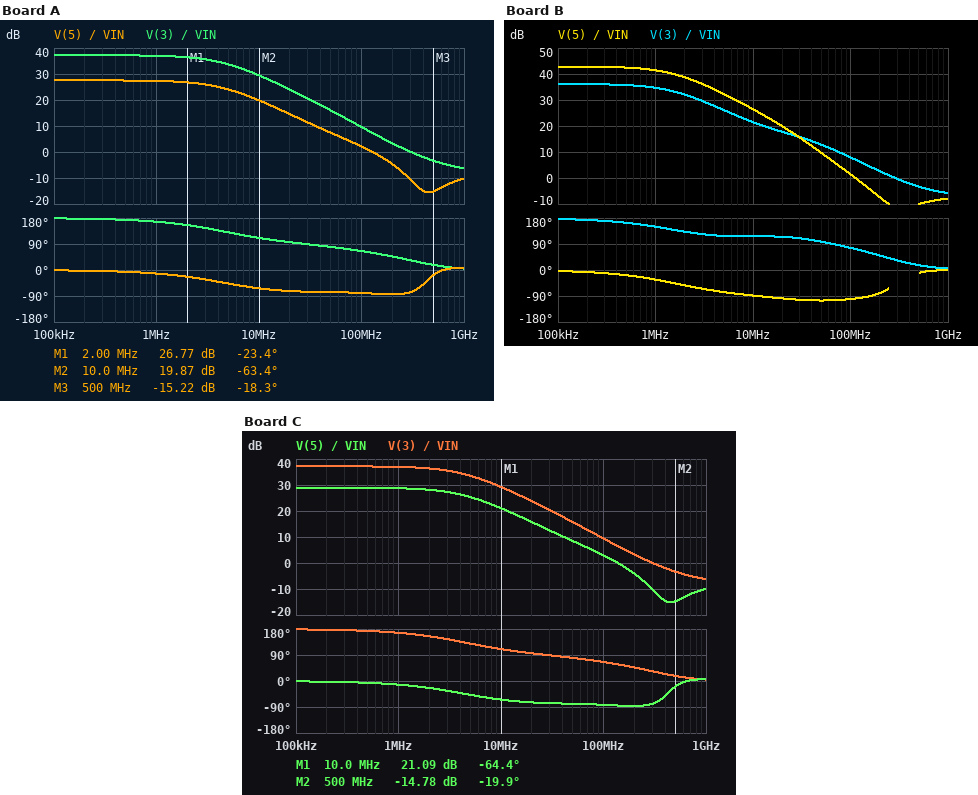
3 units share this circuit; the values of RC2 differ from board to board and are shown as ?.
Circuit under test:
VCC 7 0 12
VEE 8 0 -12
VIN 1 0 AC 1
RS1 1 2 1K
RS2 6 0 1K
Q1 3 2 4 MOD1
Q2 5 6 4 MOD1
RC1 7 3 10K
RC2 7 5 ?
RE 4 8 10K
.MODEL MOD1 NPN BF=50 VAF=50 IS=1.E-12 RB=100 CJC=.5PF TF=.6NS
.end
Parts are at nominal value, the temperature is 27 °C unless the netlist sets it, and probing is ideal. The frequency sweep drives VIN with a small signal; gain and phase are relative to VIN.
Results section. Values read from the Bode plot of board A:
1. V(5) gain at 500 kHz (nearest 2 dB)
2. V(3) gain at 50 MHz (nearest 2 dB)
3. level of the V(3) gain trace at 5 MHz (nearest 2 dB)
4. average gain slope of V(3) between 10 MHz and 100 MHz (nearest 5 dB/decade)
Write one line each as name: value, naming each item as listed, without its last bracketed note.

V(5) gain at 500 kHz: 28 dB
V(3) gain at 50 MHz: 16 dB
level of the V(3) gain trace at 5 MHz: 34 dB
average gain slope of V(3) between 10 MHz and 100 MHz: -20 dB/decade
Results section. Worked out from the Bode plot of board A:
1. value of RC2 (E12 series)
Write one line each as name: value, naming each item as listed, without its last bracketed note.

value of RC2: 3.3 kΩ
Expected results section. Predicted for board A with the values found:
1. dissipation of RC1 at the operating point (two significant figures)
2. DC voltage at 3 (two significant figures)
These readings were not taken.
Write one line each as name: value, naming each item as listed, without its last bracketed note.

dissipation of RC1 at the operating point: 3.0 mW
DC voltage at 3: 6.5 V
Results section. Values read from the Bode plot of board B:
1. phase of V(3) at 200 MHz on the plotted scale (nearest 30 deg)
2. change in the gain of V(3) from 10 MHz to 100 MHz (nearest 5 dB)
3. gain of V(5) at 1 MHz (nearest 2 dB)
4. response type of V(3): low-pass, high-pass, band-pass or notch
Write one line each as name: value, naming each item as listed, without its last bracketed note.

phase of V(3) at 200 MHz on the plotted scale: 60 deg
change in the gain of V(3) from 10 MHz to 100 MHz: -15 dB
gain of V(5) at 1 MHz: 42 dB
response type of V(3): low-pass, high-pass, band-pass or notch: low-pass
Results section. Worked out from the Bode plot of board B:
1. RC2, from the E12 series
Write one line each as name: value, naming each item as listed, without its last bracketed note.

RC2, from the E12 series: 22 kΩ
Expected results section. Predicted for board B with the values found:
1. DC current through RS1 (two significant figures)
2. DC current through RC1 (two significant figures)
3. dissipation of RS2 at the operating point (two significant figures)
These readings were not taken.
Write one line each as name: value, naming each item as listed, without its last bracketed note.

DC current through RS1: 11 µA
DC current through RC1: 590 µA
dissipation of RS2 at the operating point: 110 nW
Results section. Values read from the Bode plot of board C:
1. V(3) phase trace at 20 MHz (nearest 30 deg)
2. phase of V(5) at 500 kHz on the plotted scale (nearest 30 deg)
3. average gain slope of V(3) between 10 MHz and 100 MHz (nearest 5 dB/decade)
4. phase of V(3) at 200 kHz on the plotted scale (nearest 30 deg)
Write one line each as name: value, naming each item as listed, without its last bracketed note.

V(3) phase trace at 20 MHz: 90 deg
phase of V(5) at 500 kHz on the plotted scale: 0 deg
average gain slope of V(3) between 10 MHz and 100 MHz: -20 dB/decade
phase of V(3) at 200 kHz on the plotted scale: 180 deg
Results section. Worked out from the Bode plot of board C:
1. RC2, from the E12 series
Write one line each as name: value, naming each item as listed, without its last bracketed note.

RC2, from the E12 series: 3.9 kΩ
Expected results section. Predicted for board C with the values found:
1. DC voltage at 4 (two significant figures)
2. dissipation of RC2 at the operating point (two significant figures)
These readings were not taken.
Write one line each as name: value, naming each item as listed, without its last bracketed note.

DC voltage at 4: -530 mV
dissipation of RC2 at the operating point: 1.3 mW
